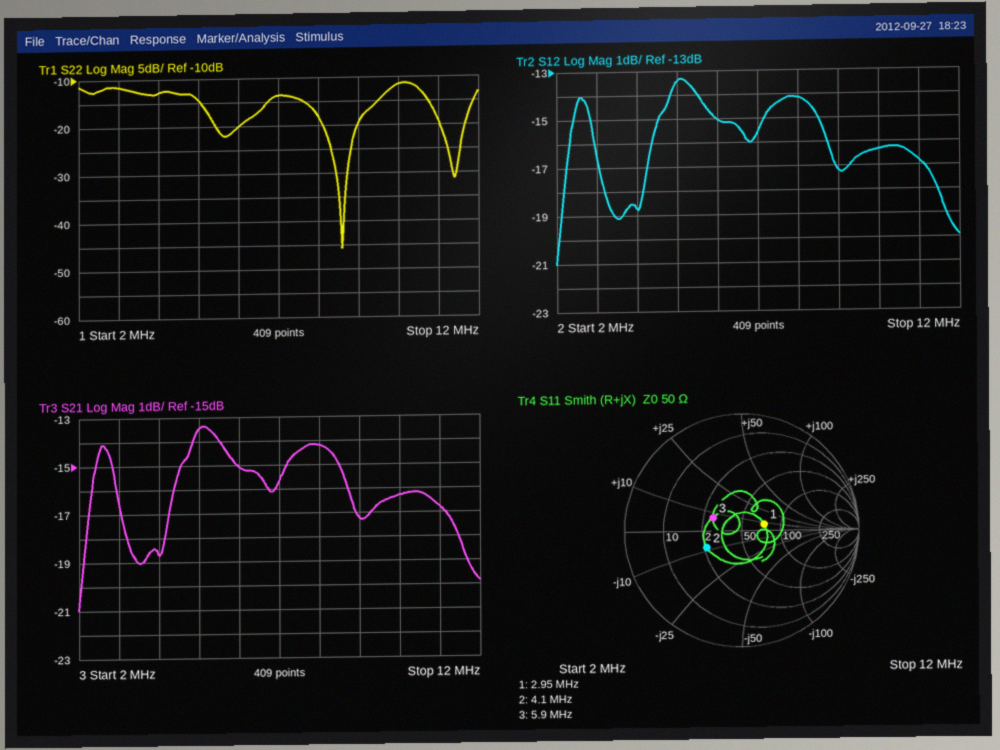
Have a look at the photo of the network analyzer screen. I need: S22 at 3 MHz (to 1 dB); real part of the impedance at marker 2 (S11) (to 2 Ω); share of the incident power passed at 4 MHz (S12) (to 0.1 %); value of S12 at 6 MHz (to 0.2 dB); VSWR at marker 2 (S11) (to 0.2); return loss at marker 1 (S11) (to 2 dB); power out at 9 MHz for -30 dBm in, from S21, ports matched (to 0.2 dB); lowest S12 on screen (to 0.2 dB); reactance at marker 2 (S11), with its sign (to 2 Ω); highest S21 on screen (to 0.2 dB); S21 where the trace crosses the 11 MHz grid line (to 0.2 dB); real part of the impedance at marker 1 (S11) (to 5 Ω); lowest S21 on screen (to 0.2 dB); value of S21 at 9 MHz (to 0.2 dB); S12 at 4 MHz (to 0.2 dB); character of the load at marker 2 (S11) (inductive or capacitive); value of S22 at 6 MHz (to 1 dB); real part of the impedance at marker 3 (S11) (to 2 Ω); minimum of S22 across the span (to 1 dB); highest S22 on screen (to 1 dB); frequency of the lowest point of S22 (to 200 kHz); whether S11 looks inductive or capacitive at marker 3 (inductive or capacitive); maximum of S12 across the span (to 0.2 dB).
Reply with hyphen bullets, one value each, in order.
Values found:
- -12 dB
- 26 Ω
- 1.3 %
- -15.0 dB
- 2.0
- 14 dB
- -47.2 dBm
- -21.0 dB
- -8 Ω
- -13.4 dB
- -16.8 dB
- 75 Ω
- -21.0 dB
- -17.2 dB
- -18.8 dB
- capacitive
- -20 dB
- 30 Ω
- -46 dB
- -11 dB
- 8.6 MHz
- inductive
- -13.4 dB
